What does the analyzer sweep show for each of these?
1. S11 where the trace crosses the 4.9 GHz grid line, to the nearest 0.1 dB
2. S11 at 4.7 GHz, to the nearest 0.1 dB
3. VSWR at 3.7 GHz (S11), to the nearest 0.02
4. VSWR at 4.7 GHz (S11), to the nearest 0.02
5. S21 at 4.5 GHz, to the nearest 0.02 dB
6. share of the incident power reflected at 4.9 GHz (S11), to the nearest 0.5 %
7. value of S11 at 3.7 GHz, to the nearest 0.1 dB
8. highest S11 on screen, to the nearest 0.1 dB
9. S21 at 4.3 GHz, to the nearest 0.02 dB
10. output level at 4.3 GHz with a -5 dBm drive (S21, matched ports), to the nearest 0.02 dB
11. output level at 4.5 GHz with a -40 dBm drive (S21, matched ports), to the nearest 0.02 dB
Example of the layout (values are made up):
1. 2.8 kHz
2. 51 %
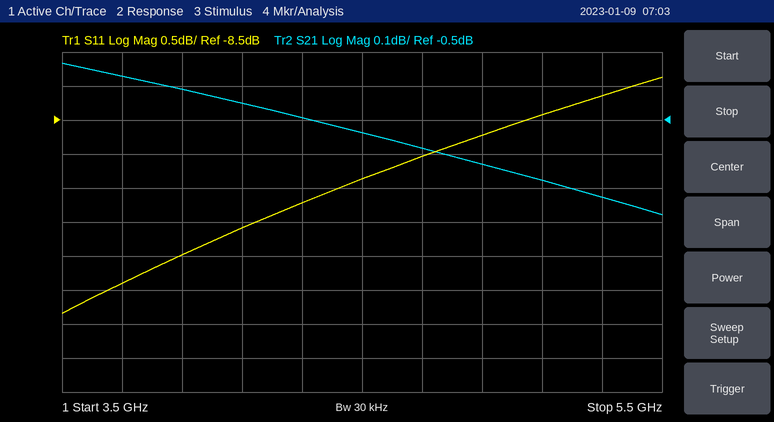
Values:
1. -8.7 dB
2. -9.0 dB
3. 1.80
4. 2.10
5. -0.54 dB
6. 13.5 %
7. -10.9 dB
8. -7.9 dB
9. -0.50 dB
10. -5.50 dBm
11. -40.54 dBm
